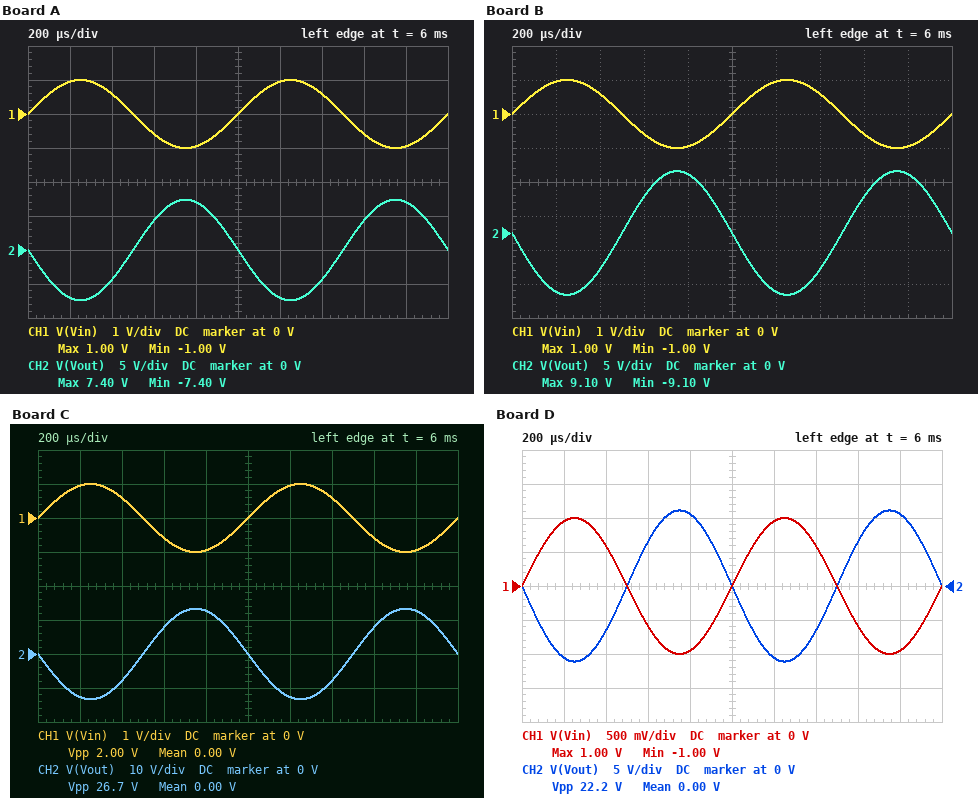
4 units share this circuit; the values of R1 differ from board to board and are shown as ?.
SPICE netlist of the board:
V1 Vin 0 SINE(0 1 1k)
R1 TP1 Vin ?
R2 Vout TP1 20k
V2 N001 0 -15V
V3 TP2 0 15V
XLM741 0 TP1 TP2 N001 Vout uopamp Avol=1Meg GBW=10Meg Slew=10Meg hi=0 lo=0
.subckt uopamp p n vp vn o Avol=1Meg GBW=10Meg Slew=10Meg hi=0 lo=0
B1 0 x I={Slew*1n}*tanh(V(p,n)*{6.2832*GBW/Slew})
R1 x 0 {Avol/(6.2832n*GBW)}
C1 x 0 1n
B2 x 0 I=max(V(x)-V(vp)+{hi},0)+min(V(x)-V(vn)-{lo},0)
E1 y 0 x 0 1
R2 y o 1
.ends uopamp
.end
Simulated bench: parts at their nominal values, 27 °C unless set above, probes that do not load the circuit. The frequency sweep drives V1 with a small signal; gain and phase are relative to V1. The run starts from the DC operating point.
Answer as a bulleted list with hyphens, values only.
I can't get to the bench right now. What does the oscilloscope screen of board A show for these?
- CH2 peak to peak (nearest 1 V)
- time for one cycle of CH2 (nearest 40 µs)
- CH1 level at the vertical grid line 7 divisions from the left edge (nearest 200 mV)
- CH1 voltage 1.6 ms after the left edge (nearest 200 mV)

- 15 V
- 1.00 ms
- 600 mV
- -600 mV
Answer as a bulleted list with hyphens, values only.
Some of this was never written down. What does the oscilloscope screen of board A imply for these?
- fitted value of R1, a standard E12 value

- 2.7 kΩ
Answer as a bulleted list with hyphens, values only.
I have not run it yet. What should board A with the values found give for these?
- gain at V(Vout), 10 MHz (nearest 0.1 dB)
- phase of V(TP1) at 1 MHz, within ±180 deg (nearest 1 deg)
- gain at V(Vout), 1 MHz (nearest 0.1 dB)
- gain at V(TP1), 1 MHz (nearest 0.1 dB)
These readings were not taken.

- -1.2 dB
- 50 deg
- 15.1 dB
- -4.9 dB
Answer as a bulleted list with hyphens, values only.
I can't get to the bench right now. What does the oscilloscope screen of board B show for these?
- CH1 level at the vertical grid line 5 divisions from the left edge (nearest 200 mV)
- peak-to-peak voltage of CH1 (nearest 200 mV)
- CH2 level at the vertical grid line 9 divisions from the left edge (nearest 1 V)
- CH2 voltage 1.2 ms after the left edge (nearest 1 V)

- 0 V
- 2.0 V
- 9 V
- -9 V
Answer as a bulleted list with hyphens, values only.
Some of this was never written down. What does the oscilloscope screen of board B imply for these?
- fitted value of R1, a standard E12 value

- 2.2 kΩ
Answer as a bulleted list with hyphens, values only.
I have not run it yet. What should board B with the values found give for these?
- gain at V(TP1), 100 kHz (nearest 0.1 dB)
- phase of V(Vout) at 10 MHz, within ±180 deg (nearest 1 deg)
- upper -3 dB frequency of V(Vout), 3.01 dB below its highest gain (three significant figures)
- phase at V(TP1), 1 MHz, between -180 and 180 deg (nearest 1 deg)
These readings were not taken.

- -20.9 dB
- 96 deg
- 991 kHz
- 45 deg
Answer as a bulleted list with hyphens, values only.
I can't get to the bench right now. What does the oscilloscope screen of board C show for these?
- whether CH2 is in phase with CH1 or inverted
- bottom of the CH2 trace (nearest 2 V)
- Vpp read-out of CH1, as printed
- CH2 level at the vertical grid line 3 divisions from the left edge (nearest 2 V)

- inverted
- -14 V
- 2.00 V
- 8 V
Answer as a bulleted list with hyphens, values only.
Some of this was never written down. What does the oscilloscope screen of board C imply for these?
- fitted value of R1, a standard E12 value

- 1.5 kΩ
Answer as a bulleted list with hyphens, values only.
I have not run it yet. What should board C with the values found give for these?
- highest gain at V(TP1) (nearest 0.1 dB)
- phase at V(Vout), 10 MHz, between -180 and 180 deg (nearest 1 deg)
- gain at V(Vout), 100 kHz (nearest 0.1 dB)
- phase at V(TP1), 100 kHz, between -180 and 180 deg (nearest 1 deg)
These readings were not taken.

- -0.6 dB
- 94 deg
- 22.4 dB
- 82 deg
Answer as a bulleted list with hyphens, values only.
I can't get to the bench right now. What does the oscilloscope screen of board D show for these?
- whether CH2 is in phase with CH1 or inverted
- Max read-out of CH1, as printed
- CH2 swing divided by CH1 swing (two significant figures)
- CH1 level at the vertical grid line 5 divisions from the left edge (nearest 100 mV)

- inverted
- 1.00 V
- 11
- 0 V
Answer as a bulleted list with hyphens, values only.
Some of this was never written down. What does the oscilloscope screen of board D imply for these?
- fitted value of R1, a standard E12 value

- 1.8 kΩ
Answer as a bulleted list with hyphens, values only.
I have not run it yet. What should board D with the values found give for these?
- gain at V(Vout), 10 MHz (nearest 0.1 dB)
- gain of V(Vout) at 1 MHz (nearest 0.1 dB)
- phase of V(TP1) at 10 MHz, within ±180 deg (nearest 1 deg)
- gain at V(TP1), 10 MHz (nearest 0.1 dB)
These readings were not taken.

- -0.8 dB
- 17.0 dB
- 5 deg
- -0.8 dB
